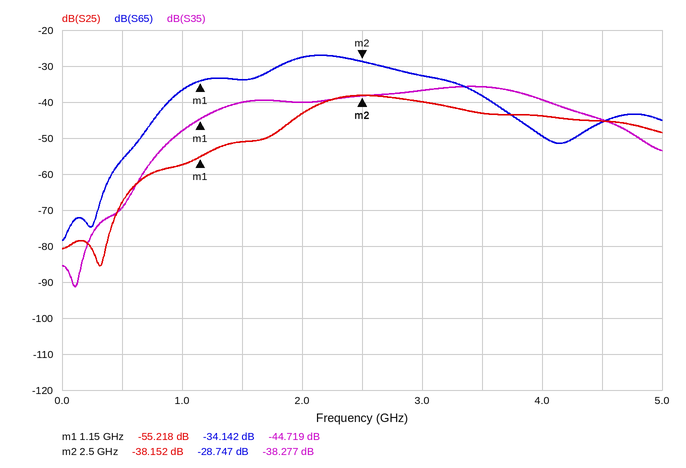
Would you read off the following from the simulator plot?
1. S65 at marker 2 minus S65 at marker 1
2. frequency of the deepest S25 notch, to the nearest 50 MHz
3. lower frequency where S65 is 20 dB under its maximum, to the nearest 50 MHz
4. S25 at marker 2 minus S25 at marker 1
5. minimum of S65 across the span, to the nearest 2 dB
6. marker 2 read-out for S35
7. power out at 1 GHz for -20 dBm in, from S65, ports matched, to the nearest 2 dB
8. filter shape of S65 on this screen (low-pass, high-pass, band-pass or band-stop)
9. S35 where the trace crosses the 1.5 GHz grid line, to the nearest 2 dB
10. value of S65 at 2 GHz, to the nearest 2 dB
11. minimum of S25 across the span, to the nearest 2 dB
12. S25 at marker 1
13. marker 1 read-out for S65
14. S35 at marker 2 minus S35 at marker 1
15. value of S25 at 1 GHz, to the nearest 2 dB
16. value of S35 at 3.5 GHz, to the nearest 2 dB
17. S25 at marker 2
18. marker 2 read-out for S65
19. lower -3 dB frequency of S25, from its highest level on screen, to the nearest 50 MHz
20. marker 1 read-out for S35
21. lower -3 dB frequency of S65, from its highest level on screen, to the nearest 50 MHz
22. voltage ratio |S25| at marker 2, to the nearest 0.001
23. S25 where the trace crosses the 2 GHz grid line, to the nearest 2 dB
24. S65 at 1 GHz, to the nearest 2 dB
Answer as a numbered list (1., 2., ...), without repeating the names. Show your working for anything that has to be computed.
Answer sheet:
1. -28.747 − (-34.142) = 5.395 dB
2. 300 MHz
3. 700 MHz
4. -38.152 − (-55.218) = 17.066 dB
5. -78 dB
6. -38.277 dB
7. -20 dBm + (-36 dB) = -56 dBm
8. band-pass
9. -40 dB
10. -28 dB
11. -86 dB
12. -55.218 dB
13. -34.142 dB
14. -38.277 − (-44.719) = 6.442 dB
15. -58 dB
16. -36 dB
17. -38.152 dB
18. -28.747 dB
19. 2.10 GHz
20. -44.719 dB
21. 1.80 GHz
22. 10^(-38.152/20) ≈ 0.012
23. -44 dB
24. -36 dB
